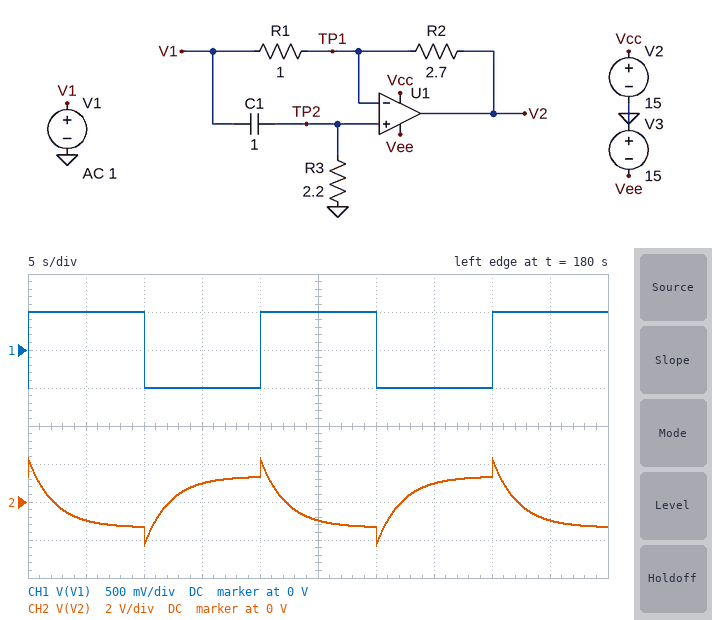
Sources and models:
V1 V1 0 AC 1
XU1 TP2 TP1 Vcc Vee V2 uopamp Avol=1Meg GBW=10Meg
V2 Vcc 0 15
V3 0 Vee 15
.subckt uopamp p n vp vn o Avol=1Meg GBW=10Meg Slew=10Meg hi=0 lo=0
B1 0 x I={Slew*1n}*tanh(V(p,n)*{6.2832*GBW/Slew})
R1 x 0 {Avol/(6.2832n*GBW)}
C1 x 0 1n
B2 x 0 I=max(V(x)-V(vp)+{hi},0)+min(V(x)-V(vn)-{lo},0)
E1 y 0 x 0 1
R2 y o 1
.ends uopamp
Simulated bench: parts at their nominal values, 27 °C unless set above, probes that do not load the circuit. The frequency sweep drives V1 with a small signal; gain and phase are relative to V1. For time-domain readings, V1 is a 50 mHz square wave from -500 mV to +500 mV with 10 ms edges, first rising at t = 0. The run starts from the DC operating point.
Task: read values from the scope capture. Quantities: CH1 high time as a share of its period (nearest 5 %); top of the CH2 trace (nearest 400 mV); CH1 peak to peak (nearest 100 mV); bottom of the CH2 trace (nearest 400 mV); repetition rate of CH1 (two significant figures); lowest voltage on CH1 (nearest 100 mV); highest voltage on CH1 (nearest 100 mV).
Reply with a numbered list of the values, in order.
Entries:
1. 50 %
2. 2.4 V
3. 1.0 V
4. -2.4 V
5. 50 mHz
6. -500 mV
7. 500 mV
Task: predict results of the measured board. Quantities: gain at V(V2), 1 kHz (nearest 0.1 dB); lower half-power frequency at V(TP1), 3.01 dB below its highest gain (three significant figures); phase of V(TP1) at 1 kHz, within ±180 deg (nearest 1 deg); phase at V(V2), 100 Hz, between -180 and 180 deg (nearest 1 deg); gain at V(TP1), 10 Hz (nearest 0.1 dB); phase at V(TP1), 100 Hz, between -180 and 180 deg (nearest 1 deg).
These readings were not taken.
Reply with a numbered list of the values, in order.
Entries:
1. 0 dB
2. 72.3 mHz
3. 0 deg
4. 0 deg
5. 0 dB
6. 0 deg
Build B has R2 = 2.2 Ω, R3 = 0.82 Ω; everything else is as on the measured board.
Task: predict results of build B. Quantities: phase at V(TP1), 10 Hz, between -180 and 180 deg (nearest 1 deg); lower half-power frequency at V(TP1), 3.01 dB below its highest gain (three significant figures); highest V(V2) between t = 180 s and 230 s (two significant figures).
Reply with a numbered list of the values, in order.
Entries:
1. 1 deg
2. 194 mHz
3. 2.1 V
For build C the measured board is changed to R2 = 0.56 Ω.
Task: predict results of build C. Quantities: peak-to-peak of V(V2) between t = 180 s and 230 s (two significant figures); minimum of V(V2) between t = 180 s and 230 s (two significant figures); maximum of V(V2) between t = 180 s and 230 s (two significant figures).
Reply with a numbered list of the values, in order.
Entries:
1. 2.5 V
2. -1.3 V
3. 1.3 V
